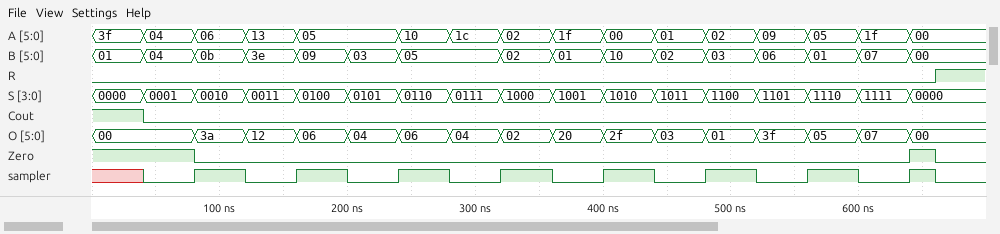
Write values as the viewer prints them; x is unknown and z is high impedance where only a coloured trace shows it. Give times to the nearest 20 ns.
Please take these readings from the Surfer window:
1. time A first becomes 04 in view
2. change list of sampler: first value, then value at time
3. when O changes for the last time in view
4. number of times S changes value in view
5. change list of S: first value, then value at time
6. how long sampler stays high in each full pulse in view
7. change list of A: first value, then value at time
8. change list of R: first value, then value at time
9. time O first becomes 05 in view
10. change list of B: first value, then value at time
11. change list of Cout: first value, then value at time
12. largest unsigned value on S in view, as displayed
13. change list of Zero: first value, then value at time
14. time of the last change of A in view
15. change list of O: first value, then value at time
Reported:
40 ns
x, 0 at 40 ns, 1 at 80 ns, 0 at 120 ns, 1 at 160 ns, 0 at 200 ns, 1 at 240 ns, 0 at 280 ns, 1 at 320 ns, 0 at 360 ns, 1 at 400 ns, 0 at 440 ns, 1 at 480 ns, 0 at 520 ns, 1 at 560 ns, 0 at 600 ns, 1 at 640 ns, 0 at 660 ns
640 ns
16
0000, 0001 at 40 ns, 0010 at 80 ns, 0011 at 120 ns, 0100 at 160 ns, 0101 at 200 ns, 0110 at 240 ns, 0111 at 280 ns, 1000 at 320 ns, 1001 at 360 ns, 1010 at 400 ns, 1011 at 440 ns, 1100 at 480 ns, 1101 at 520 ns, 1110 at 560 ns, 1111 at 600 ns, 0000 at 640 ns
40 ns, 40 ns, 40 ns, 40 ns, 40 ns, 40 ns, 40 ns, 20 ns
3f, 04 at 40 ns, 06 at 80 ns, 13 at 120 ns, 05 at 160 ns, 10 at 240 ns, 1c at 280 ns, 02 at 320 ns, 1f at 360 ns, 00 at 400 ns, 01 at 440 ns, 02 at 480 ns, 09 at 520 ns, 05 at 560 ns, 1f at 600 ns, 00 at 640 ns
0, 1 at 660 ns
560 ns
01, 04 at 40 ns, 0b at 80 ns, 3e at 120 ns, 09 at 160 ns, 03 at 200 ns, 05 at 240 ns, 02 at 320 ns, 01 at 360 ns, 10 at 400 ns, 02 at 440 ns, 03 at 480 ns, 06 at 520 ns, 01 at 560 ns, 07 at 600 ns, 00 at 640 ns
1, 0 at 40 ns
1111
1, 0 at 80 ns, 1 at 640 ns, 0 at 660 ns
640 ns
00, 3a at 80 ns, 12 at 120 ns, 06 at 160 ns, 04 at 200 ns, 06 at 240 ns, 04 at 280 ns, 02 at 320 ns, 20 at 360 ns, 2f at 400 ns, 03 at 440 ns, 01 at 480 ns, 3f at 520 ns, 05 at 560 ns, 07 at 600 ns, 00 at 640 ns
